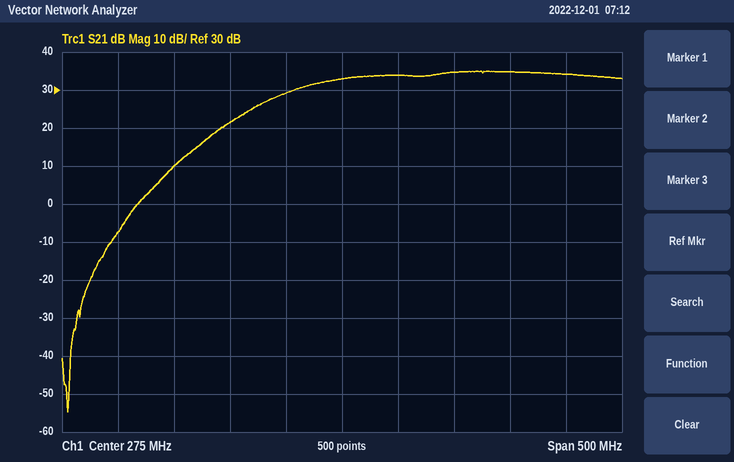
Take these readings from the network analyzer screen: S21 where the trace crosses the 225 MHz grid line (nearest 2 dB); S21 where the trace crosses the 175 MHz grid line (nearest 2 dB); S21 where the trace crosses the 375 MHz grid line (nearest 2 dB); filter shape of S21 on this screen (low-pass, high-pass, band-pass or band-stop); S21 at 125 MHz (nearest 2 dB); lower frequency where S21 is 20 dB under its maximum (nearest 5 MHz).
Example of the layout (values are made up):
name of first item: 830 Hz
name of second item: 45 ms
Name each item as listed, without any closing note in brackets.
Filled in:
S21 where the trace crosses the 225 MHz grid line: 30 dB
S21 where the trace crosses the 175 MHz grid line: 22 dB
S21 where the trace crosses the 375 MHz grid line: 34 dB
filter shape of S21 on this screen: high-pass
S21 at 125 MHz: 10 dB
lower frequency where S21 is 20 dB under its maximum: 145 MHz
